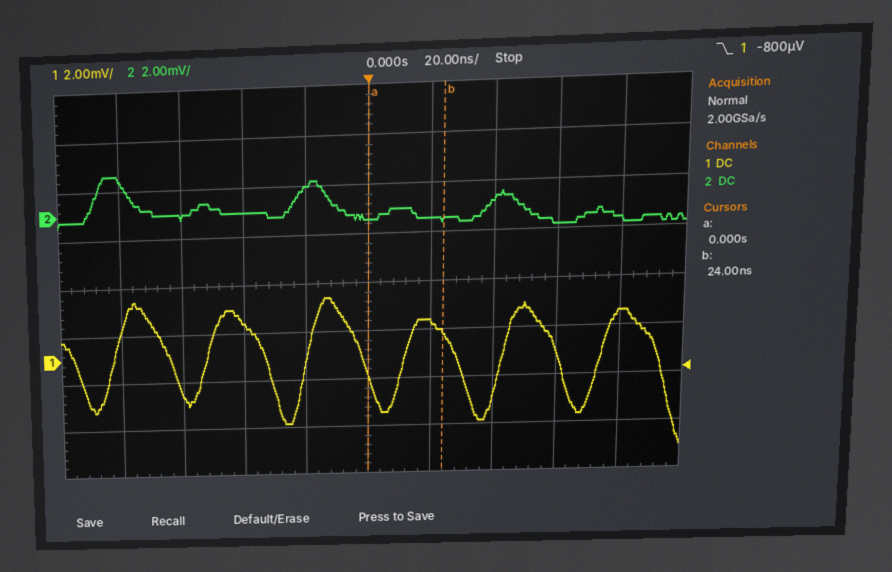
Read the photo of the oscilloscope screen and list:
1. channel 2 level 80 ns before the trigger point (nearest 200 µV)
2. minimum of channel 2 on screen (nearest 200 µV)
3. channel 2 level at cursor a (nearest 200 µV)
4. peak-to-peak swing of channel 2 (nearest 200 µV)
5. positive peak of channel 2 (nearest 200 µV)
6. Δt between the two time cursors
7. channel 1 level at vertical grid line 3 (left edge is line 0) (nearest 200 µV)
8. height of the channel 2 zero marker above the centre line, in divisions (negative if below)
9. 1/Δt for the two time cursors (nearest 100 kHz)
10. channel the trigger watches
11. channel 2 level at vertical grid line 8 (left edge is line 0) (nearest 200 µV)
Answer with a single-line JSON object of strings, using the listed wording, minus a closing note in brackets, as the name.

{"channel 2 level 80 ns before the trigger point": "1.4 mV", "minimum of channel 2 on screen": "-800 µV", "channel 2 level at cursor a": "-400 µV", "peak-to-peak swing of channel 2": "2.4 mV", "positive peak of channel 2": "1.6 mV", "Δt between the two time cursors": "24 ns", "channel 1 level at vertical grid line 3 (left edge is line 0)": "1.4 mV", "height of the channel 2 zero marker above the centre line, in divisions": "+1.5 div", "1/Δt for the two time cursors": "41.7 MHz", "channel the trigger watches": "channel 1", "channel 2 level at vertical grid line 8 (left edge is line 0)": "-800 µV"}
